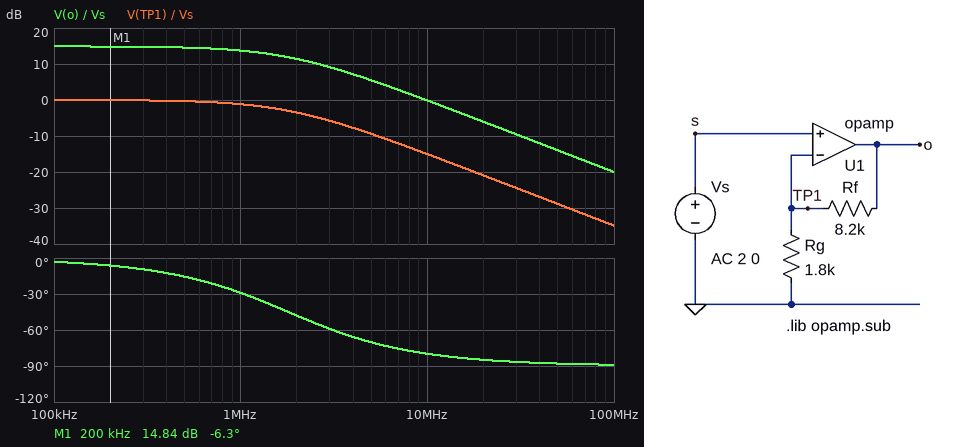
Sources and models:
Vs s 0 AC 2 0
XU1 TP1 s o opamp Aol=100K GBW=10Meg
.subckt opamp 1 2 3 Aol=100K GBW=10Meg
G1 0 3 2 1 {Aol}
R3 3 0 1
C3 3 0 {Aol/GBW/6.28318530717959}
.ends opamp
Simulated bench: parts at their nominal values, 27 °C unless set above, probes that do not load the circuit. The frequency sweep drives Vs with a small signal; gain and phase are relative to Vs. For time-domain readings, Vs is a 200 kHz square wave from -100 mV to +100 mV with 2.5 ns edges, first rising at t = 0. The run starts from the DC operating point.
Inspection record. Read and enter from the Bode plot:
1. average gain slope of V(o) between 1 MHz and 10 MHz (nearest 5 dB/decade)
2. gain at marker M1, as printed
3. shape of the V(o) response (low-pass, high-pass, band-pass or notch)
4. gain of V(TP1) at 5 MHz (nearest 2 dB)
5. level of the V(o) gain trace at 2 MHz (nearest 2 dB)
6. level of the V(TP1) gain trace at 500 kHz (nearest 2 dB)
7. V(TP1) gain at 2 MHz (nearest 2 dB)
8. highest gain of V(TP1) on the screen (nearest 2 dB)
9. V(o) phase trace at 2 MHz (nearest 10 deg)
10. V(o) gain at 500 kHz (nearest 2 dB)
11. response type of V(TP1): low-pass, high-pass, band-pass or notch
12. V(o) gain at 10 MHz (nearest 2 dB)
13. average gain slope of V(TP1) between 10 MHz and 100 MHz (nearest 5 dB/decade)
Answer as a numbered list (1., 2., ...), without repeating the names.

1. -15 dB/decade
2. 14.84 dB
3. low-pass
4. -10 dB
5. 12 dB
6. 0 dB
7. -4 dB
8. 0 dB
9. -50 deg
10. 14 dB
11. low-pass
12. 0 dB
13. -20 dB/decade
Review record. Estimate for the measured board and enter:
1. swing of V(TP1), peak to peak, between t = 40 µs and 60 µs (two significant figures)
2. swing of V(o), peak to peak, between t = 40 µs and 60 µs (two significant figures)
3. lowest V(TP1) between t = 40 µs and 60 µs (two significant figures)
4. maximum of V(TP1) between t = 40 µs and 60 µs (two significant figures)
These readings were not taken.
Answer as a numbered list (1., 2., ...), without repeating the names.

1. 200 mV
2. 1.1 V
3. -100 mV
4. 100 mV
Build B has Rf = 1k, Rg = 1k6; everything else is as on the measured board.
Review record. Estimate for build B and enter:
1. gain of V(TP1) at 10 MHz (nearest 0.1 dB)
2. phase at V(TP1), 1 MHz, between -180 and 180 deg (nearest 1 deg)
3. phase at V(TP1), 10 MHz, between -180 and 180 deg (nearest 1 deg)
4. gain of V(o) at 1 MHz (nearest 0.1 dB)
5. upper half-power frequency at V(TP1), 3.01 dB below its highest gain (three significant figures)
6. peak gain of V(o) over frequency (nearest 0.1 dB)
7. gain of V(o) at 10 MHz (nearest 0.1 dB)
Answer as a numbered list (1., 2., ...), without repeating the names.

1. -5.6 dB
2. -9 deg
3. -58 deg
4. 4.1 dB
5. 6.15 MHz
6. 4.2 dB
7. -1.4 dB
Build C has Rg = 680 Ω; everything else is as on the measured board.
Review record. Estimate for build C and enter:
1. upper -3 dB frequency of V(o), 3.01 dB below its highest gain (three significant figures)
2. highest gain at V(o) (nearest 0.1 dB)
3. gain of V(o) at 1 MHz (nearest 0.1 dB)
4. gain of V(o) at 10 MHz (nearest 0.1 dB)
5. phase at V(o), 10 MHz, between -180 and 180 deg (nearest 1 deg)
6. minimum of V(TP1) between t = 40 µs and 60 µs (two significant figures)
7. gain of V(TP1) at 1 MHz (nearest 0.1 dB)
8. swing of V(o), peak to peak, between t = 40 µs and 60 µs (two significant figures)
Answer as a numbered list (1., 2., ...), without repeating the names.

1. 766 kHz
2. 22.3 dB
3. 18.0 dB
4. 0 dB
5. -86 deg
6. -100 mV
7. -4.3 dB
8. 2.6 V
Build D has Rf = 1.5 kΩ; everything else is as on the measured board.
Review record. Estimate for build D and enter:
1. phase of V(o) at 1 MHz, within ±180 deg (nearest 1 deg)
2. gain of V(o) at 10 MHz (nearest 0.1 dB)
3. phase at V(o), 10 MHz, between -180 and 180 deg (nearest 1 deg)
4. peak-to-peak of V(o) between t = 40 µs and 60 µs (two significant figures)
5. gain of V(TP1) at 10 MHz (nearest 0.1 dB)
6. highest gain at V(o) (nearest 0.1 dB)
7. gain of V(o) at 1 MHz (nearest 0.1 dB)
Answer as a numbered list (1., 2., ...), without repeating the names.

1. -10 deg
2. -1.1 dB
3. -61 deg
4. 370 mV
5. -6.4 dB
6. 5.3 dB
7. 5.1 dB
